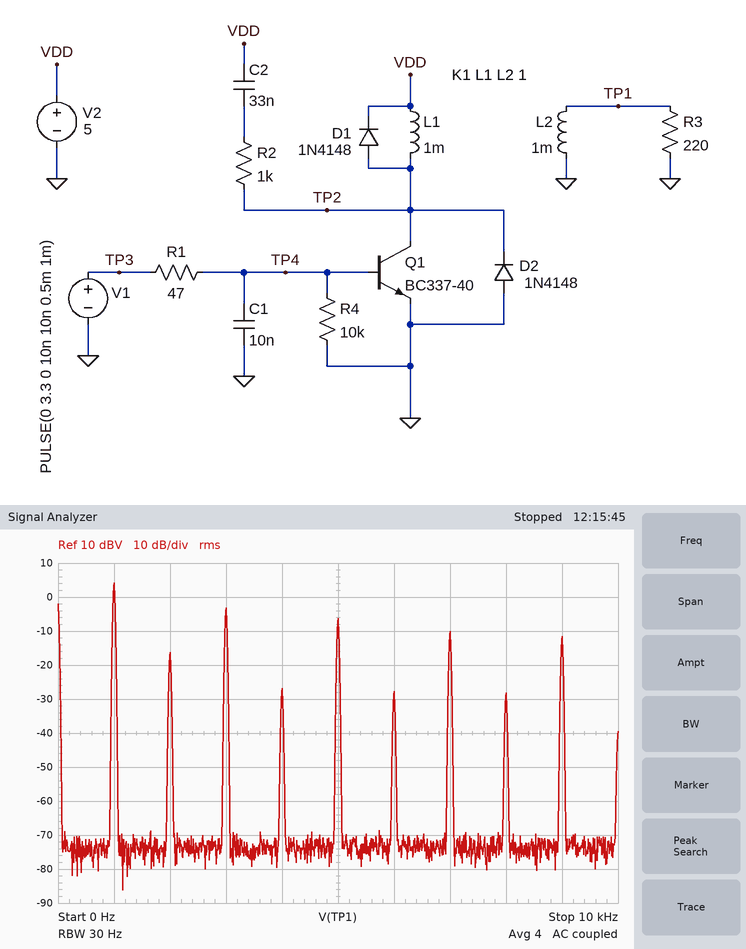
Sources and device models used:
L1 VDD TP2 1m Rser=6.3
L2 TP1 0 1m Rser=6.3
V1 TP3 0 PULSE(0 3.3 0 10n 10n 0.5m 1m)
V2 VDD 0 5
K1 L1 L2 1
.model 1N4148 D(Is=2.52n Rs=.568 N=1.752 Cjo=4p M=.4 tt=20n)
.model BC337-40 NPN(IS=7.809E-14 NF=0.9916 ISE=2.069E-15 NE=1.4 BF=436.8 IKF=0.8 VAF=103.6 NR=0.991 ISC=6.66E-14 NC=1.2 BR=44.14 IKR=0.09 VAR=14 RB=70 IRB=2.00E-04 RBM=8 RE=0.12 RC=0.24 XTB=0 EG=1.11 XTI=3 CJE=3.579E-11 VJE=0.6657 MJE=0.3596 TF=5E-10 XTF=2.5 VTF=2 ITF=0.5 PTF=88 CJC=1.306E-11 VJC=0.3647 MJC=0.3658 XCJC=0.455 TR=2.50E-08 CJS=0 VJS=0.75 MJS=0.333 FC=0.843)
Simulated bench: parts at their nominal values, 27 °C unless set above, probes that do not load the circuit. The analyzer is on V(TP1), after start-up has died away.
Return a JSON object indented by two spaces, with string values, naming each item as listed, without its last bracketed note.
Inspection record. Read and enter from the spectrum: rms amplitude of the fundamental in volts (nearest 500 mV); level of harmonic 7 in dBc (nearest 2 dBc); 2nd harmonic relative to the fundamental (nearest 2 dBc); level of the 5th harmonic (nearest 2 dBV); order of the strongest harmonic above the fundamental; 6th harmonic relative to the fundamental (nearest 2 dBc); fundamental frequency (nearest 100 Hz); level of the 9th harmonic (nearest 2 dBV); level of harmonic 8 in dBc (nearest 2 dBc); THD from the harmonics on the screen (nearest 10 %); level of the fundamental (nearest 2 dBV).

{
  "rms amplitude of the fundamental in volts": "1.5 V",
  "level of harmonic 7 in dBc": "-14 dBc",
  "2nd harmonic relative to the fundamental": "-20 dBc",
  "level of the 5th harmonic": "-6 dBV",
  "order of the strongest harmonic above the fundamental": "3",
  "6th harmonic relative to the fundamental": "-32 dBc",
  "fundamental frequency": "1.0 kHz",
  "level of the 9th harmonic": "-12 dBV",
  "level of harmonic 8 in dBc": "-32 dBc",
  "THD from the harmonics on the screen": "60 %",
  "level of the fundamental": "4 dBV"
}
